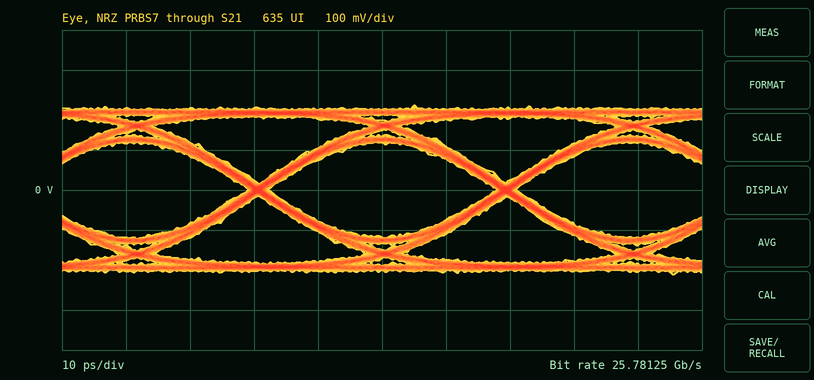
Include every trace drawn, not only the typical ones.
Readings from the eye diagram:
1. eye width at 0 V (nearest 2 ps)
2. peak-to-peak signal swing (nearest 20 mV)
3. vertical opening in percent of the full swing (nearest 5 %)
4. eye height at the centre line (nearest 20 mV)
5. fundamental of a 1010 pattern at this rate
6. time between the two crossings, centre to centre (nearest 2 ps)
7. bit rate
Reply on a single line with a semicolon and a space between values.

36 ps; 420 mV; 55 %; 240 mV; 12.89062 GHz; 38 ps; 25.78125 Gb/s
